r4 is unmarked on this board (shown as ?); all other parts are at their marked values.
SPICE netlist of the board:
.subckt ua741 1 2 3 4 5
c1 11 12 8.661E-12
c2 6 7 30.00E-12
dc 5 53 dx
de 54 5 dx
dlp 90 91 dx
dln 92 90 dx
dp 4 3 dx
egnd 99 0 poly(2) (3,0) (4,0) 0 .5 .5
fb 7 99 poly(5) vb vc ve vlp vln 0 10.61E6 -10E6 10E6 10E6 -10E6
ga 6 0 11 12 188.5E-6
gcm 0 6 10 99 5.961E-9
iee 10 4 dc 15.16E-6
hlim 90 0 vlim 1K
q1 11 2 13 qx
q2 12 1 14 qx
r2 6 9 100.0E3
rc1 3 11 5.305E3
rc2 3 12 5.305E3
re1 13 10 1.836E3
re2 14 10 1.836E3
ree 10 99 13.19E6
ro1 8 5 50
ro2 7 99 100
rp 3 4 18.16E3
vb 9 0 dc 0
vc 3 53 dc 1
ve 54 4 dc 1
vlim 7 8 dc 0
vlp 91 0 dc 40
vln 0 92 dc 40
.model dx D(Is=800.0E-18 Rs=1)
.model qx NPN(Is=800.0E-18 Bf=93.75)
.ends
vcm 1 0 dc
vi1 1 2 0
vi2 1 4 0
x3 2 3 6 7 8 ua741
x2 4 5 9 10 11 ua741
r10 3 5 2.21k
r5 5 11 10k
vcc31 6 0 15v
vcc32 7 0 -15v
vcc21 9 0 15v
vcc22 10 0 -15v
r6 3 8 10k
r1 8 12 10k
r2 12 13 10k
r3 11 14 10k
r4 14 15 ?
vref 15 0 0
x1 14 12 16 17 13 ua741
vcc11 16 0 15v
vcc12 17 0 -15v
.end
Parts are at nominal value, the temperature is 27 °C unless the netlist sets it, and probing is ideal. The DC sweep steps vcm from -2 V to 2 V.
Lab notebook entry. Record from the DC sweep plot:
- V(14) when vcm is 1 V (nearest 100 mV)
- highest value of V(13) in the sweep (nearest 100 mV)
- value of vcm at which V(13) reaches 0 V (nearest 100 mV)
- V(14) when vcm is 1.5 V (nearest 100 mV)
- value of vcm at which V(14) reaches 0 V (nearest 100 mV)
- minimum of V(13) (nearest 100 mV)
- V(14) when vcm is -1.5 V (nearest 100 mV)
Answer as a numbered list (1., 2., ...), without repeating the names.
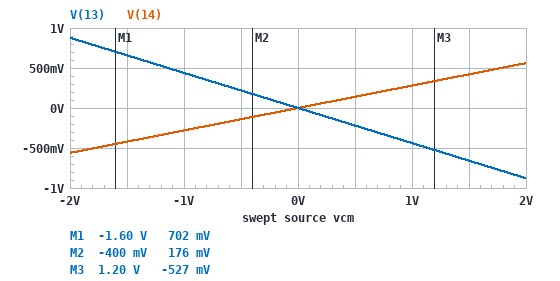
1. 300 mV
2. 900 mV
3. 0 V
4. 400 mV
5. 0 V
6. -900 mV
7. -400 mV
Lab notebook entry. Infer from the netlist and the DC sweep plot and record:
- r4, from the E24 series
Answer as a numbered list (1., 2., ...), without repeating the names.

1. 3.9 kΩ
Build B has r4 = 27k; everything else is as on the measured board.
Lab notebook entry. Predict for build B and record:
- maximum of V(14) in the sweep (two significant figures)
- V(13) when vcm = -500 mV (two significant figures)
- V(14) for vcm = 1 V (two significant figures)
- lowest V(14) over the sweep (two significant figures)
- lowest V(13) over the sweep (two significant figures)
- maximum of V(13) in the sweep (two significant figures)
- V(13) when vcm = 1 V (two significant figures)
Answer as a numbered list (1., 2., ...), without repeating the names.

1. 1.5 V
2. -230 mV
3. 730 mV
4. -1.5 V
5. -920 mV
6. 920 mV
7. 460 mV
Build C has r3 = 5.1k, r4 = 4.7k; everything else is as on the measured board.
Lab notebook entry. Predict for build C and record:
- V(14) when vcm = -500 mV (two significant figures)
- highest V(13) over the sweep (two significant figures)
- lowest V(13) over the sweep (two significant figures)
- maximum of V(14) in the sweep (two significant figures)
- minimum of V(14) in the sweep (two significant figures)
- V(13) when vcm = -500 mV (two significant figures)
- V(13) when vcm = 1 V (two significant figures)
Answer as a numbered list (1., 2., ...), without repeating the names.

1. -240 mV
2. 82 mV
3. -81 mV
4. 960 mV
5. -960 mV
6. 21 mV
7. -40 mV
